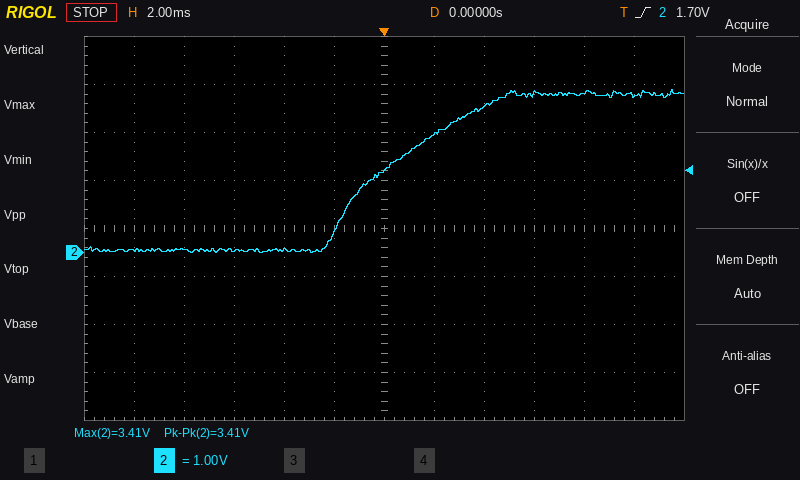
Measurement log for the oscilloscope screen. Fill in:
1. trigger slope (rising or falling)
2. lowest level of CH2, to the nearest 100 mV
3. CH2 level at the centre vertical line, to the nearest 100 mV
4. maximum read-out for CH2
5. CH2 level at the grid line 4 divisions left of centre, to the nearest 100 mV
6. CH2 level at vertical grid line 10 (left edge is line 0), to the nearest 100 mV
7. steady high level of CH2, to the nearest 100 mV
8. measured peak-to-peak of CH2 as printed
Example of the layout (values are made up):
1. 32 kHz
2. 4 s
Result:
1. rising
2. 0.0 V
3. 1.7 V
4. 3.41 V
5. 100 mV
6. 3.3 V
7. 3.3 V
8. 3.41 V
